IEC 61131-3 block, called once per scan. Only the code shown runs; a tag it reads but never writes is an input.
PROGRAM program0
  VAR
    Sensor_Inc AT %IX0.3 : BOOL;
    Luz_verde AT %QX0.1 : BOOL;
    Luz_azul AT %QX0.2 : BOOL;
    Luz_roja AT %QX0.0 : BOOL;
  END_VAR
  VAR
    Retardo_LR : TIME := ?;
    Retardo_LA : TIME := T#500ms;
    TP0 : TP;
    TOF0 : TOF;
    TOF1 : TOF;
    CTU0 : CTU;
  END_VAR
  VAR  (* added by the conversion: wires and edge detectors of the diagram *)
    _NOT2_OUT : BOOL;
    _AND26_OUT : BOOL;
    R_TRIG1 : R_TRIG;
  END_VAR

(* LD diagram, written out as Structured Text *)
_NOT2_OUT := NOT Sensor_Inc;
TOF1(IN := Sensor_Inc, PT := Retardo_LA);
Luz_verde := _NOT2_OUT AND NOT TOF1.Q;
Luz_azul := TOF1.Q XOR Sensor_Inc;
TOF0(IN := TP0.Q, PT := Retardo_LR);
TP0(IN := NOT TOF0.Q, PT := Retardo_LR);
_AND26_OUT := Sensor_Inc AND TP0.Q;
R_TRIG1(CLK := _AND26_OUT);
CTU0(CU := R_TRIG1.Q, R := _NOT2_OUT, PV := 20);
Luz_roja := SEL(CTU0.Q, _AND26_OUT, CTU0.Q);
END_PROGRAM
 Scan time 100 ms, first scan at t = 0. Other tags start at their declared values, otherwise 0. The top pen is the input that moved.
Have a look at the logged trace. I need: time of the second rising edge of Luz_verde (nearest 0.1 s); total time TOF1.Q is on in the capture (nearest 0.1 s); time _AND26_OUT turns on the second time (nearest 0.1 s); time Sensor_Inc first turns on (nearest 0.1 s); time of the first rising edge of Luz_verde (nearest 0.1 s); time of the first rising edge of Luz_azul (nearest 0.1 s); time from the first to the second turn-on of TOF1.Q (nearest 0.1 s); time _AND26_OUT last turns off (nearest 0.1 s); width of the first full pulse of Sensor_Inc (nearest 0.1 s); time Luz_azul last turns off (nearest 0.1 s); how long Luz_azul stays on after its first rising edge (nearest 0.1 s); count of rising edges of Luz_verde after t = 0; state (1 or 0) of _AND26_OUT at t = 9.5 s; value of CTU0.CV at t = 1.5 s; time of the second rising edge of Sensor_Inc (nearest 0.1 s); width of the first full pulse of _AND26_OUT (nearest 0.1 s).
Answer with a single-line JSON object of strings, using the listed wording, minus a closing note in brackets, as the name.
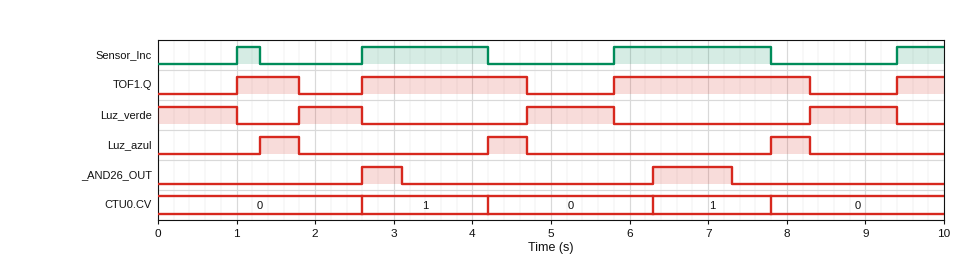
{"time of the second rising edge of Luz_verde": "4.7 s", "total time TOF1.Q is on in the capture": "6.0 s", "time _AND26_OUT turns on the second time": "6.3 s", "time Sensor_Inc first turns on": "1.0 s", "time of the first rising edge of Luz_verde": "1.8 s", "time of the first rising edge of Luz_azul": "1.3 s", "time from the first to the second turn-on of TOF1.Q": "1.6 s", "time _AND26_OUT last turns off": "7.3 s", "width of the first full pulse of Sensor_Inc": "0.3 s", "time Luz_azul last turns off": "8.3 s", "how long Luz_azul stays on after its first rising edge": "0.5 s", "count of rising edges of Luz_verde after t = 0": "3", "state (1 or 0) of _AND26_OUT at t = 9.5 s": "0", "value of CTU0.CV at t = 1.5 s": "0", "time of the second rising edge of Sensor_Inc": "2.6 s", "width of the first full pulse of _AND26_OUT": "0.5 s"}
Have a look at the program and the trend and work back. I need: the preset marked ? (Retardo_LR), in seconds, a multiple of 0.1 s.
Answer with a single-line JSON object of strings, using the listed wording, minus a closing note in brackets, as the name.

{"the preset marked ? (Retardo_LR), in seconds, a multiple of 0.1 s": "1.0 s"}
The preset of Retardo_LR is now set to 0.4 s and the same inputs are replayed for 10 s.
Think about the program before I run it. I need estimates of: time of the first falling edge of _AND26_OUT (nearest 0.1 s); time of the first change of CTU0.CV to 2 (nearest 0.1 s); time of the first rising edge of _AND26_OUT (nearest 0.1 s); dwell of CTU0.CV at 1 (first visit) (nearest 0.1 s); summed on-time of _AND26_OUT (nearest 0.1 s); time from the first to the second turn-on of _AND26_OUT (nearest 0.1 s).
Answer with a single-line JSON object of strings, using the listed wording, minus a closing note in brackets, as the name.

{"time of the first falling edge of _AND26_OUT": "1.3 s", "time of the first change of CTU0.CV to 2": "3.6 s", "time of the first rising edge of _AND26_OUT": "1.0 s", "dwell of CTU0.CV at 1 (first visit)": "0.3 s", "summed on-time of _AND26_OUT": "2.0 s", "time from the first to the second turn-on of _AND26_OUT": "1.7 s"}
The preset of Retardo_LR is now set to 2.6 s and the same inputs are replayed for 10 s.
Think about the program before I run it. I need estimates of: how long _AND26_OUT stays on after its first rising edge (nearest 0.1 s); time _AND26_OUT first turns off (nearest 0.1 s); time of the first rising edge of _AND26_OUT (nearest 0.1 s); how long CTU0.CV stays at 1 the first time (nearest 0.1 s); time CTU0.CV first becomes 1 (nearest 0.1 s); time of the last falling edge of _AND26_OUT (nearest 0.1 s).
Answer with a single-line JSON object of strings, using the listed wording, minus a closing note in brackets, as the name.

{"how long _AND26_OUT stays on after its first rising edge": "0.3 s", "time _AND26_OUT first turns off": "1.3 s", "time of the first rising edge of _AND26_OUT": "1.0 s", "how long CTU0.CV stays at 1 the first time": "0.3 s", "time CTU0.CV first becomes 1": "1.0 s", "time of the last falling edge of _AND26_OUT": "7.8 s"}
